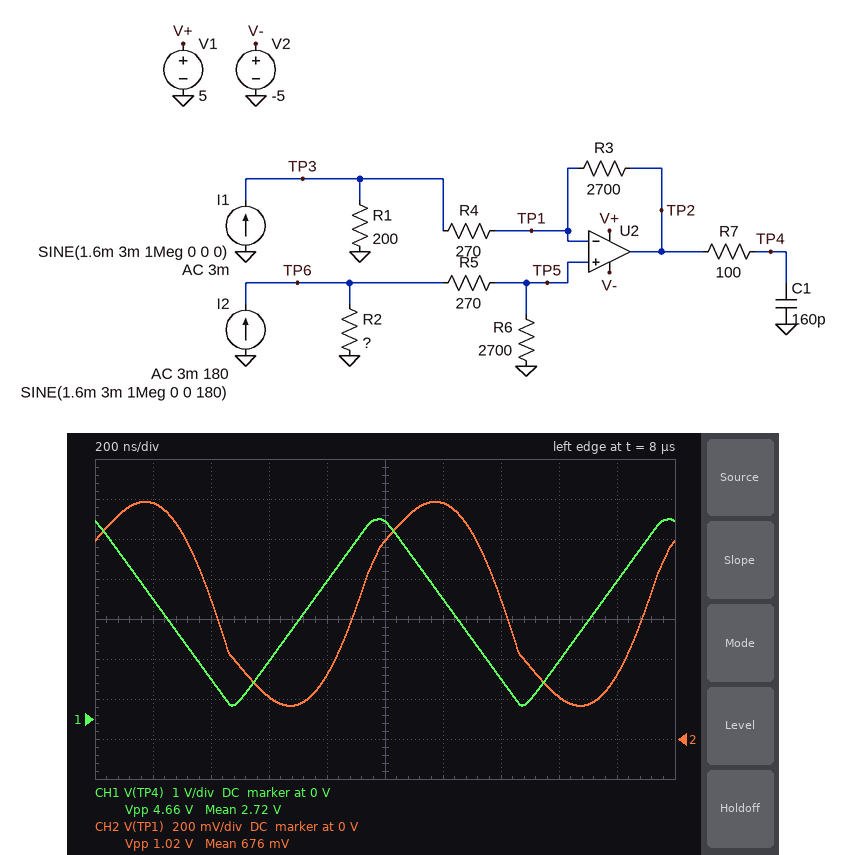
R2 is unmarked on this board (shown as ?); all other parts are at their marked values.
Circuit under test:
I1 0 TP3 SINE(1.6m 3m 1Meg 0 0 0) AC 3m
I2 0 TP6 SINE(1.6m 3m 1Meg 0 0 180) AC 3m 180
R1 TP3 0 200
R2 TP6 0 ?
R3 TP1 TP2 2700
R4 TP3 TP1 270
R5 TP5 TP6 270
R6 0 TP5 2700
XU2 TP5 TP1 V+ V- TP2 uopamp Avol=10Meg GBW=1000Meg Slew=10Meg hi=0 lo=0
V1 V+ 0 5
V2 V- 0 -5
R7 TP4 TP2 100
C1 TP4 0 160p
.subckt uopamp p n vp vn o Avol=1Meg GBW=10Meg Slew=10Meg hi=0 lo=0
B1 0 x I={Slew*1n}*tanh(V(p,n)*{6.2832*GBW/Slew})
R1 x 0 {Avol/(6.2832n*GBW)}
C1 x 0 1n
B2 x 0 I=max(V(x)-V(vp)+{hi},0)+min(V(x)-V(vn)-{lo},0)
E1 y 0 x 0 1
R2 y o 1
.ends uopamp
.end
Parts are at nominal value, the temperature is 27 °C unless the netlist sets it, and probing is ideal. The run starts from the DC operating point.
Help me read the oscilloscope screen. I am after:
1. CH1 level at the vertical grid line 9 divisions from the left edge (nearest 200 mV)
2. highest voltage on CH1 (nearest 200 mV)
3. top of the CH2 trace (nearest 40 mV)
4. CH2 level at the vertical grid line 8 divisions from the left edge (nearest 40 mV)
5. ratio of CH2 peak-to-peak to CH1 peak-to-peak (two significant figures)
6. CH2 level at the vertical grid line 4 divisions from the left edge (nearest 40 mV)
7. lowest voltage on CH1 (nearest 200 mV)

3.4 V
5.0 V
1.20 V
200 mV
0.22
320 mV
400 mV
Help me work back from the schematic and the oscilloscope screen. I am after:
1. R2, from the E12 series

680 Ω
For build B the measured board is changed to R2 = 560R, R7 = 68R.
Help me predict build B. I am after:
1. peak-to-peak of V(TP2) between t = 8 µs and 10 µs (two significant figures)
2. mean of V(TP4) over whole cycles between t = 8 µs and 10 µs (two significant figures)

4.9 V
2.6 V
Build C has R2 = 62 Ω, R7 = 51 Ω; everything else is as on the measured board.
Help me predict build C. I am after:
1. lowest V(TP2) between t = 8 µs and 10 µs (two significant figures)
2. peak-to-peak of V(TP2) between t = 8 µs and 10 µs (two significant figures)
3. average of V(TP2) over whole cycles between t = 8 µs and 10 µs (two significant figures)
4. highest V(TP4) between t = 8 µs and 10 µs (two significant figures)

-3.7 V
5.0 V
-1.2 V
1.2 V
